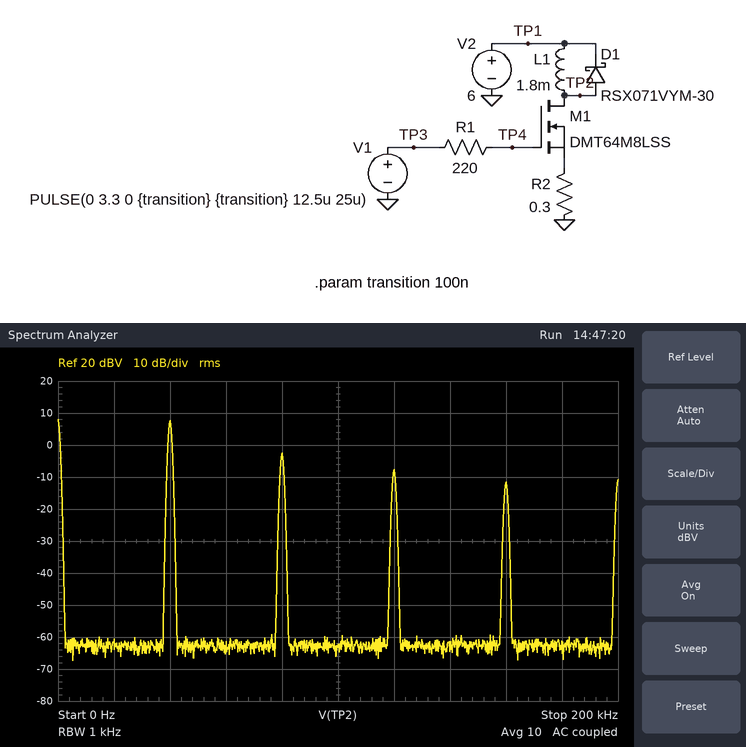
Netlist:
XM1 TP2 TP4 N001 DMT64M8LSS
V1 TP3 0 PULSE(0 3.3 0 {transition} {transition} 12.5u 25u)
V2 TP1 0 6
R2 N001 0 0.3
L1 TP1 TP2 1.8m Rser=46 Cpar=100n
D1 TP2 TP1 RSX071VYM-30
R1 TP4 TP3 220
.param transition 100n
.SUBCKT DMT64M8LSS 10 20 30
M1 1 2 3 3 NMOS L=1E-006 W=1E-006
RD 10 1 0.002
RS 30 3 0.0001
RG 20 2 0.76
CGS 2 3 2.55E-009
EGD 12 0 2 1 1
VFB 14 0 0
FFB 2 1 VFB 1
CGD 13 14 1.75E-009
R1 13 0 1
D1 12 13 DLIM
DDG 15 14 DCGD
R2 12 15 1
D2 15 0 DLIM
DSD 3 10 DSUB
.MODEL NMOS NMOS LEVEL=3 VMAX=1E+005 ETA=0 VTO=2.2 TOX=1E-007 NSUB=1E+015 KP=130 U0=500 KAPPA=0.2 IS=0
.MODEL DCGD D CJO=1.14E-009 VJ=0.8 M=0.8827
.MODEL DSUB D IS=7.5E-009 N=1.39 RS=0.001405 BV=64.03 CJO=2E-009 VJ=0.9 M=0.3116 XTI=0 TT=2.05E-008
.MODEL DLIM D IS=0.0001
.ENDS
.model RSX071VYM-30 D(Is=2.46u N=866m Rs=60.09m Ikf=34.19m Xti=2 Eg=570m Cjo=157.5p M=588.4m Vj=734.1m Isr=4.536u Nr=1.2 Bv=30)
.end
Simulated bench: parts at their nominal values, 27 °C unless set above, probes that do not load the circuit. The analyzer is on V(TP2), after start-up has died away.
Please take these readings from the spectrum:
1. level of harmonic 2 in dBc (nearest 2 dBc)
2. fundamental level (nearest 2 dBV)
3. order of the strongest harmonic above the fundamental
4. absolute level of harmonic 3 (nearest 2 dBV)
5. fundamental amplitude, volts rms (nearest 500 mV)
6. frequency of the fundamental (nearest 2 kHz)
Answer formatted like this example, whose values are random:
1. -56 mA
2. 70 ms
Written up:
1. -10 dBc
2. 8 dBV
3. 2
4. -8 dBV
5. 2.5 V
6. 40 kHz
